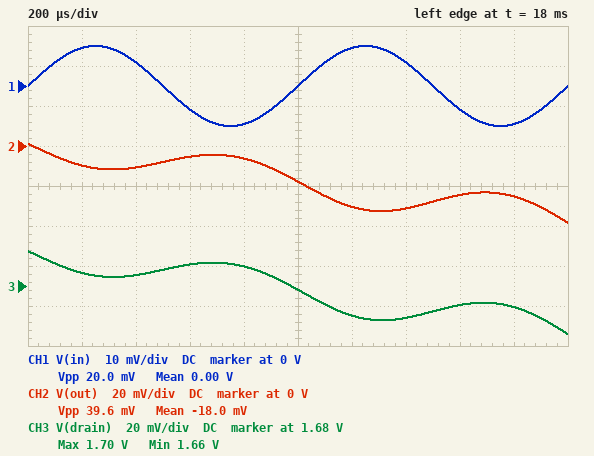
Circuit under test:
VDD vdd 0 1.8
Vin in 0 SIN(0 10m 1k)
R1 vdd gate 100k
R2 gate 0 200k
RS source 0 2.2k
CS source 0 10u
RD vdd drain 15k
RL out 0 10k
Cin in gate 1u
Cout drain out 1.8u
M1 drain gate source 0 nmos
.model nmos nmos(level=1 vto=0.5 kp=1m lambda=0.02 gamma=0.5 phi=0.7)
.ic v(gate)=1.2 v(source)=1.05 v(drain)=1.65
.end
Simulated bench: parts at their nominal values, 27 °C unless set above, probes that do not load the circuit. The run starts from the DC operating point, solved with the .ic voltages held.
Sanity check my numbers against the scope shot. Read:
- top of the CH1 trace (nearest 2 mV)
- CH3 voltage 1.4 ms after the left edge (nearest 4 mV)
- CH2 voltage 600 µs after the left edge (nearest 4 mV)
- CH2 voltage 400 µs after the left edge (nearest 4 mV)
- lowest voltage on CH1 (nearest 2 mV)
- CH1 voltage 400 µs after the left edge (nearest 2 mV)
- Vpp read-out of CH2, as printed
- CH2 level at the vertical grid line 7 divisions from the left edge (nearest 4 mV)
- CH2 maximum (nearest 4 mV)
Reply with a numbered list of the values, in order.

1. 10 mV
2. 1.664 V
3. -4 mV
4. -12 mV
5. -10 mV
6. 6 mV
7. 39.6 mV
8. -32 mV
9. 0 V
